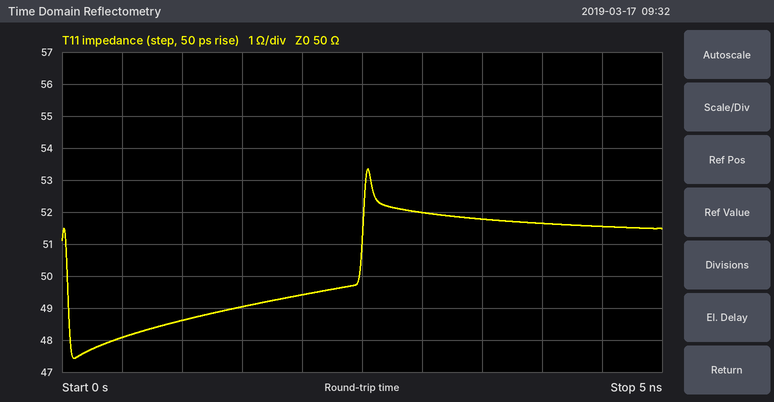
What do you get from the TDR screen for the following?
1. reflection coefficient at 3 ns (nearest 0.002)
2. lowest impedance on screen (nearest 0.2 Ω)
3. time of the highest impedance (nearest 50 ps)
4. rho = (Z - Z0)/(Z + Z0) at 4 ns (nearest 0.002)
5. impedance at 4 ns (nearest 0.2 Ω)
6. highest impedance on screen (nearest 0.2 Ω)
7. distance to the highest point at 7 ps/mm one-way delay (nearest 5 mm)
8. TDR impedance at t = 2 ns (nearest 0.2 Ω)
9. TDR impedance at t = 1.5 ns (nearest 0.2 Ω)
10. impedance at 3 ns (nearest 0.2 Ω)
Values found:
+0.020
47.4 Ω
2.55 ns
+0.016
51.6 Ω
53.4 Ω
180 mm
49.4 Ω
49.0 Ω
52.0 Ω
